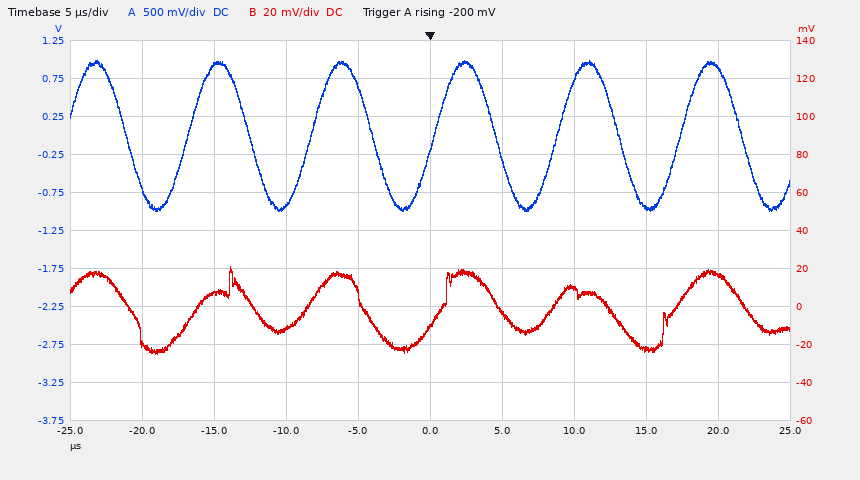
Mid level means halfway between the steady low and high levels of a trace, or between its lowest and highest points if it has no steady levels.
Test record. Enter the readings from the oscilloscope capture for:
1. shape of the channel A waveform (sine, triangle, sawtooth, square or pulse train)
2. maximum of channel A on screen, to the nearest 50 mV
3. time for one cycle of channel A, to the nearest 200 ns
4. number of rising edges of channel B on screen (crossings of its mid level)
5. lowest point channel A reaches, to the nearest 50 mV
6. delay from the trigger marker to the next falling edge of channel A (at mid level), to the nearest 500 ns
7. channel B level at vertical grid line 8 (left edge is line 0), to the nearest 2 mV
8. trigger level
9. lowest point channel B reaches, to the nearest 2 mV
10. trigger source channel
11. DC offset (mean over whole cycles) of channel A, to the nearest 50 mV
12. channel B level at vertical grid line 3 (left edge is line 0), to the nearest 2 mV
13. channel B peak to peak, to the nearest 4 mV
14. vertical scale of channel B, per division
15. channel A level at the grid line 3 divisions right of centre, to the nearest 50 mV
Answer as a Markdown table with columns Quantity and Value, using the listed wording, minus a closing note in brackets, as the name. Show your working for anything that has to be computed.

| Quantity | Value |
|---|---|
| shape of the channel A waveform | sine |
| maximum of channel A on screen, to the nearest 50 mV | 1.00 V |
| time for one cycle of channel A, to the nearest 200 ns | 8.6 µs |
| number of rising edges of channel B on screen | 5 |
| lowest point channel A reaches, to the nearest 50 mV | -1.00 V |
| delay from the trigger marker to the next falling edge of channel A (at mid level), to the nearest 500 ns | 4.5 µs |
| channel B level at vertical grid line 8 (left edge is line 0), to the nearest 2 mV | -22 mV |
| trigger level | -200 mV |
| lowest point channel B reaches, to the nearest 2 mV | -24 mV |
| trigger source channel | channel A |
| DC offset (mean over whole cycles) of channel A, to the nearest 50 mV | (1.00 V + (-1.00 V)) / 2 ≈ 0 mV |
| channel B level at vertical grid line 3 (left edge is line 0), to the nearest 2 mV | -12 mV |
| channel B peak to peak, to the nearest 4 mV | 44 mV |
| vertical scale of channel B, per division | 20 mV |
| channel A level at the grid line 3 divisions right of centre, to the nearest 50 mV | -950 mV |
